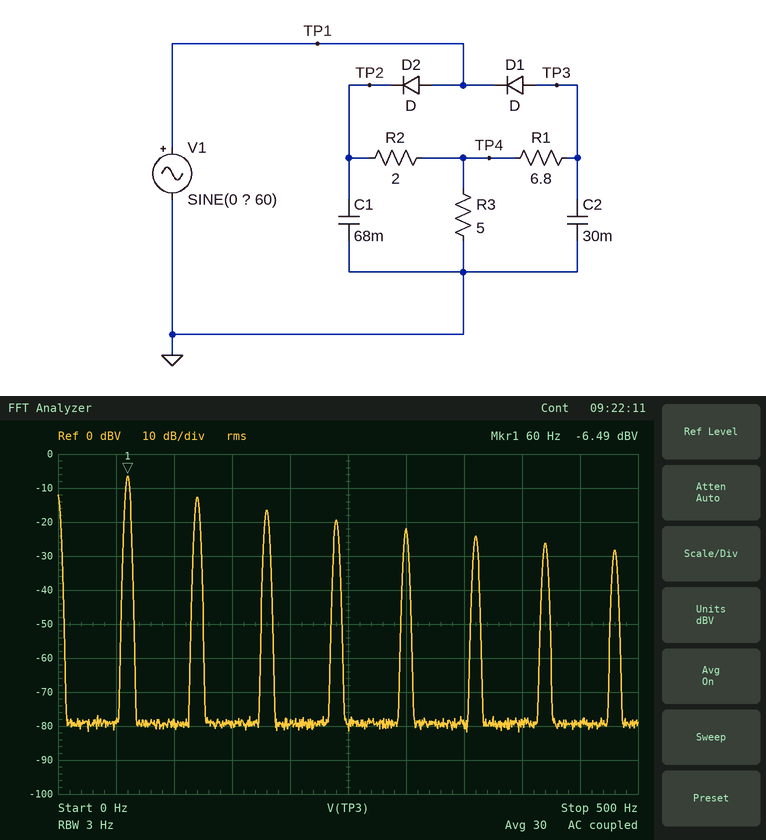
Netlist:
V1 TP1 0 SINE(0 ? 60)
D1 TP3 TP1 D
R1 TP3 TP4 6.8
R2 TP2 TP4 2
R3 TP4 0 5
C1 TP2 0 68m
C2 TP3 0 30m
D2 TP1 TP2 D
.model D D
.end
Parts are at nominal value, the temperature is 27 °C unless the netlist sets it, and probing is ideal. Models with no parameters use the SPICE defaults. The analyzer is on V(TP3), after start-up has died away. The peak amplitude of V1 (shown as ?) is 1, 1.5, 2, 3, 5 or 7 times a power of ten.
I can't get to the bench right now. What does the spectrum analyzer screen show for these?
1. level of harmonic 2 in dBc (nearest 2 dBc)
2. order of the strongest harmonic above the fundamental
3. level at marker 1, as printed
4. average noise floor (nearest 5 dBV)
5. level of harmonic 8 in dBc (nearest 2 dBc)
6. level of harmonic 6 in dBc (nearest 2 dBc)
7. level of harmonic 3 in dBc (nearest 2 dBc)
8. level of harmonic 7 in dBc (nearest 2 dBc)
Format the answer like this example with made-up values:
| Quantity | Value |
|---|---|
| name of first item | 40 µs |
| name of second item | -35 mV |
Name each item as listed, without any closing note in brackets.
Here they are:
| Quantity | Value |
|---|---|
| level of harmonic 2 in dBc | -6 dBc |
| order of the strongest harmonic above the fundamental | 2 |
| level at marker 1, as printed | -6.49 dBV |
| average noise floor | -80 dBV |
| level of harmonic 8 in dBc | -22 dBc |
| level of harmonic 6 in dBc | -18 dBc |
| level of harmonic 3 in dBc | -10 dBc |
| level of harmonic 7 in dBc | -20 dBc |
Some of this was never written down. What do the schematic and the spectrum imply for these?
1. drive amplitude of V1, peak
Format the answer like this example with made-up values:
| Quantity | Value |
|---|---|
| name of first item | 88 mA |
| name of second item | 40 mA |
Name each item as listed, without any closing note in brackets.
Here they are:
| Quantity | Value |
|---|---|
| drive amplitude of V1, peak | 20 V |
